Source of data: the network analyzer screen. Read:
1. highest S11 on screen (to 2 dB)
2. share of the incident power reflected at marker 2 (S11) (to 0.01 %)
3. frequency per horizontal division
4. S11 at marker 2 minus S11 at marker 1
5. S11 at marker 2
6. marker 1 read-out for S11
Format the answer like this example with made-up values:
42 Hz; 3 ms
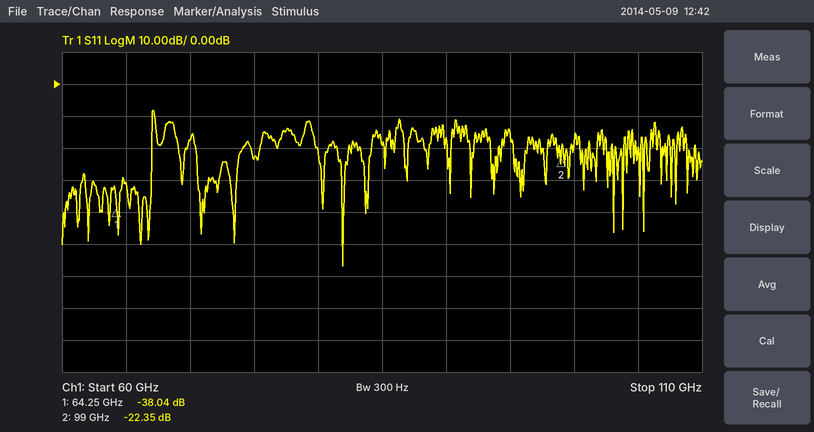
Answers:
-8 dB; 0.58 %; 5 GHz; 15.69 dB; -22.35 dB; -38.04 dB
